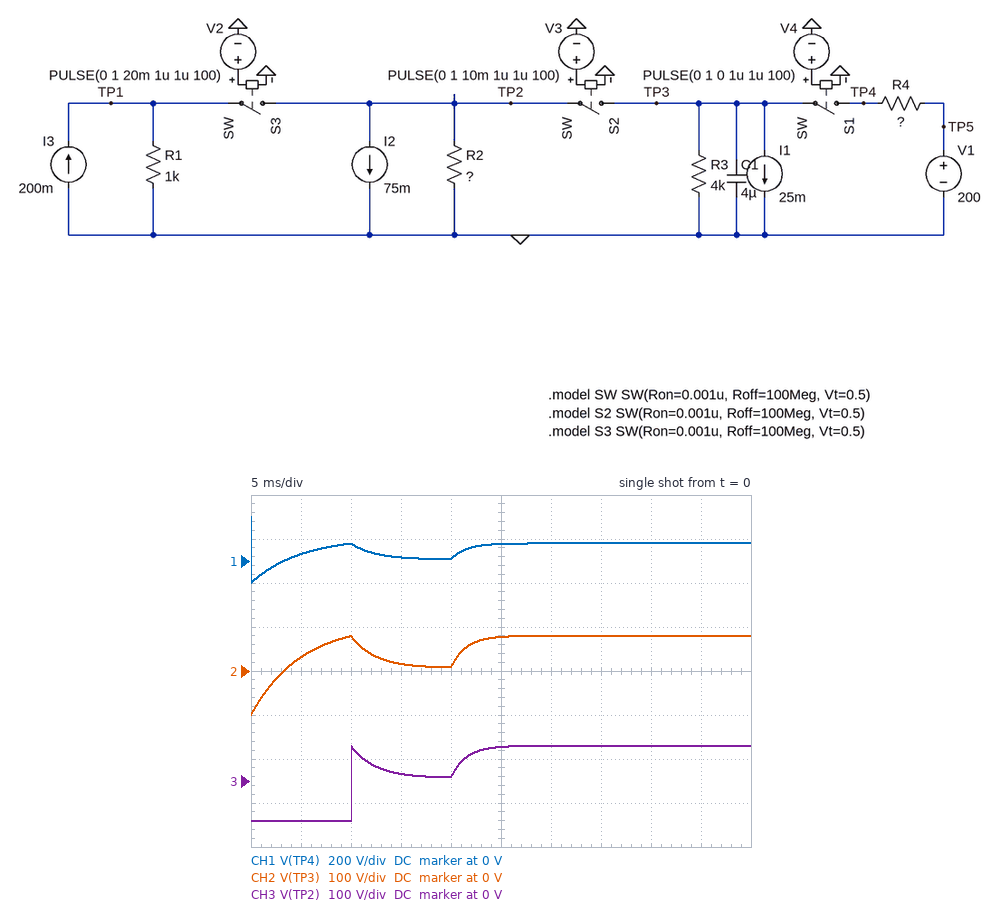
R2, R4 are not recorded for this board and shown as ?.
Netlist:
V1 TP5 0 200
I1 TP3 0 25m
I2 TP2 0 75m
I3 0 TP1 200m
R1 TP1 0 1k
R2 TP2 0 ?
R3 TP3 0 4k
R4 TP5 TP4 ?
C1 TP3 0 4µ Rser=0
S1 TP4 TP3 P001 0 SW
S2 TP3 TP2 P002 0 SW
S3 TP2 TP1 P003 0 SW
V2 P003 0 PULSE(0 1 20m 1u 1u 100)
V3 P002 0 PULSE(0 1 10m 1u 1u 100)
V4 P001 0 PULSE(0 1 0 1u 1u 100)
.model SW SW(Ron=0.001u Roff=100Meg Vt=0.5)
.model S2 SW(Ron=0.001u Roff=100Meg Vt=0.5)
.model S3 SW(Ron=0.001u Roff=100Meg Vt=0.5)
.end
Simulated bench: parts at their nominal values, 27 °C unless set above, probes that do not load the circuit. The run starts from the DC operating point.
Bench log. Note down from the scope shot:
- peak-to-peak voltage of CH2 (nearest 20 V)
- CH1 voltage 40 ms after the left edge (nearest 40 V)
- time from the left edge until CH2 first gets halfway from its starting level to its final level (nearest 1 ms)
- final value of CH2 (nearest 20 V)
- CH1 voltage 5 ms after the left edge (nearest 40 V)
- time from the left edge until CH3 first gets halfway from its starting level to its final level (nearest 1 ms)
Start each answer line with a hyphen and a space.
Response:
- 180 V
- 80 V
- 3 ms
- 80 V
- 40 V
- 10 ms
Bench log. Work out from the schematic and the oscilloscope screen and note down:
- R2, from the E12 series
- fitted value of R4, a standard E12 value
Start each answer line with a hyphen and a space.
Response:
- 1.2 kΩ
- 1.8 kΩ
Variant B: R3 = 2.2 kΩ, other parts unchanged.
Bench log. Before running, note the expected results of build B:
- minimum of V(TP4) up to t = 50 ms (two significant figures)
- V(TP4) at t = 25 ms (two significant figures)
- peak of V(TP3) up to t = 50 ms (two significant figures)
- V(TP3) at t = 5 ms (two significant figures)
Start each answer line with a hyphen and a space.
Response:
- -55 V
- 72 V
- 74 V
- 46 V
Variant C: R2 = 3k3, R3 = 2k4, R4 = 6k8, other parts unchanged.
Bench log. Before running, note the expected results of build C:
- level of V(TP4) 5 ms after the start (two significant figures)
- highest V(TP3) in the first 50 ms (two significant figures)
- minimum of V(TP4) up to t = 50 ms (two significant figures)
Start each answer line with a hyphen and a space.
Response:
- -26 V
- 69 V
- -73 V
